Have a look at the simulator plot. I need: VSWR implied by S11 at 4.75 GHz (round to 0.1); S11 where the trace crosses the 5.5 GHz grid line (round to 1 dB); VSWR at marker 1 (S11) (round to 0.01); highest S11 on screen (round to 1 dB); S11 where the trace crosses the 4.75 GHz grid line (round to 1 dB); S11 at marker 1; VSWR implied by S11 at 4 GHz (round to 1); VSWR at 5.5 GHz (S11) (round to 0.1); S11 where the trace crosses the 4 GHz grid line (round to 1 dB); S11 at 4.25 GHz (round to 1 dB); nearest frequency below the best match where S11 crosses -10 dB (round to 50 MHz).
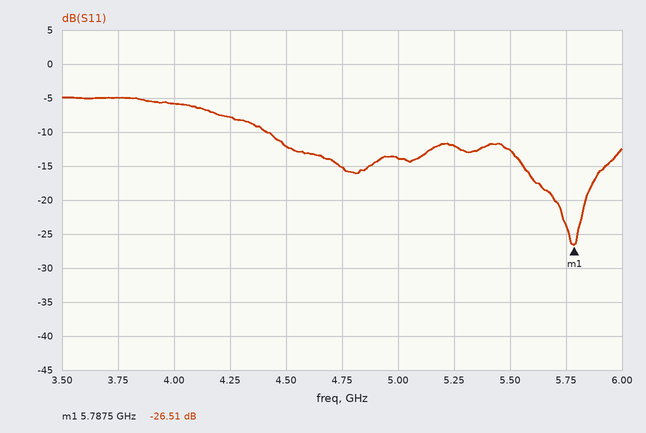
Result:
1.4
-13 dB
1.10
-5 dB
-15 dB
-26.51 dB
3
1.6
-6 dB
-8 dB
4.40 GHz
